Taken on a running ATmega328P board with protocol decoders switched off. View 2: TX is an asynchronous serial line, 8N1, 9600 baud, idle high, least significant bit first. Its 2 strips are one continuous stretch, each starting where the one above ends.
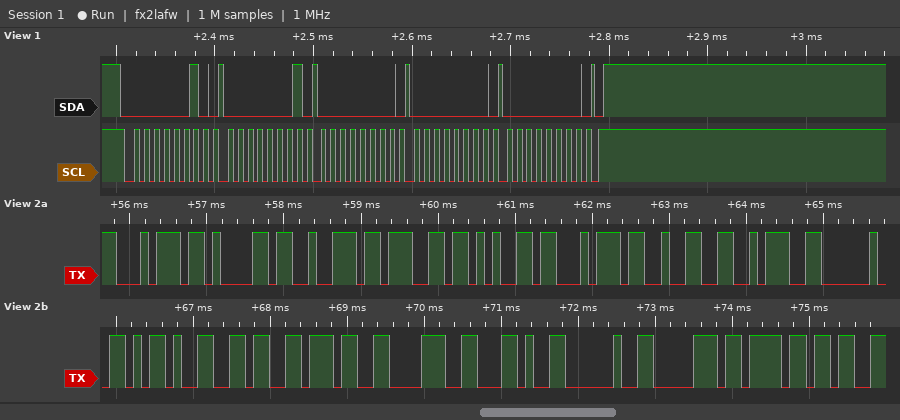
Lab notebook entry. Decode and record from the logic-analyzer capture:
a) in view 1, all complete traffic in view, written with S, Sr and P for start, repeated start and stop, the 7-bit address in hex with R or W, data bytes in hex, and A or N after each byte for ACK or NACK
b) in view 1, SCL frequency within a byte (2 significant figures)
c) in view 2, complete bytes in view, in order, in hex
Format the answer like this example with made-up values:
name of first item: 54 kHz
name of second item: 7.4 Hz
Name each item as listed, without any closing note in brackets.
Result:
in view 1, all complete traffic in view, written with S, Sr and P for start, repeated start and stop, the 7-bit address in hex with R or W, data bytes in hex, and A or N after each byte for ACK or NACK: S 01W A 01 A 00 A 00 A 00 A P
in view 1, SCL frequency within a byte: 100 kHz
in view 2, complete bytes in view, in order, in hex: 74 61 72 67 65 74 32 3A 20 2D 36 37 38 2C 20 70 6F
